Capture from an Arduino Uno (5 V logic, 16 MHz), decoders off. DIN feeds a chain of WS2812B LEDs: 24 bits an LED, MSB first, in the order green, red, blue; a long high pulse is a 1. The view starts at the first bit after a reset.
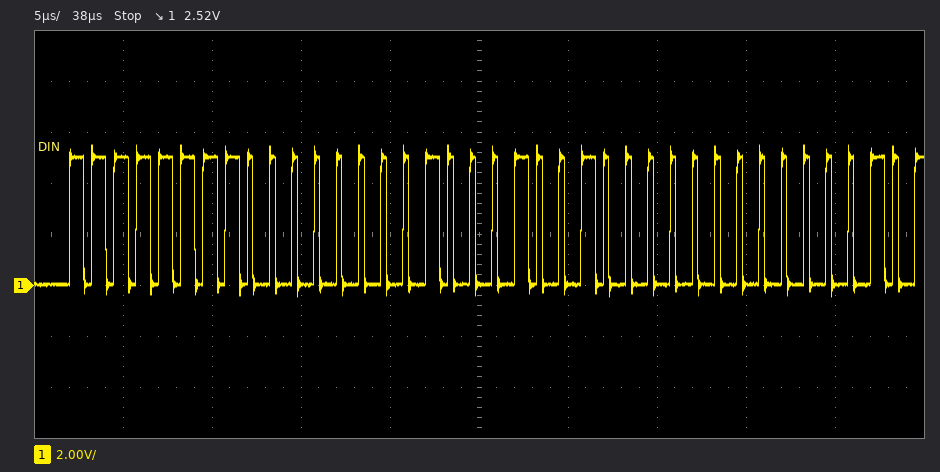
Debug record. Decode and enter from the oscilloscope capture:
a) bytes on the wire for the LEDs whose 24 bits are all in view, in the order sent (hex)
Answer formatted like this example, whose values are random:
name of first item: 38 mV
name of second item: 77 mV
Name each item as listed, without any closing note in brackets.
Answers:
bytes on the wire for the LEDs whose 24 bits are all in view, in the order sent: FF 00 89
